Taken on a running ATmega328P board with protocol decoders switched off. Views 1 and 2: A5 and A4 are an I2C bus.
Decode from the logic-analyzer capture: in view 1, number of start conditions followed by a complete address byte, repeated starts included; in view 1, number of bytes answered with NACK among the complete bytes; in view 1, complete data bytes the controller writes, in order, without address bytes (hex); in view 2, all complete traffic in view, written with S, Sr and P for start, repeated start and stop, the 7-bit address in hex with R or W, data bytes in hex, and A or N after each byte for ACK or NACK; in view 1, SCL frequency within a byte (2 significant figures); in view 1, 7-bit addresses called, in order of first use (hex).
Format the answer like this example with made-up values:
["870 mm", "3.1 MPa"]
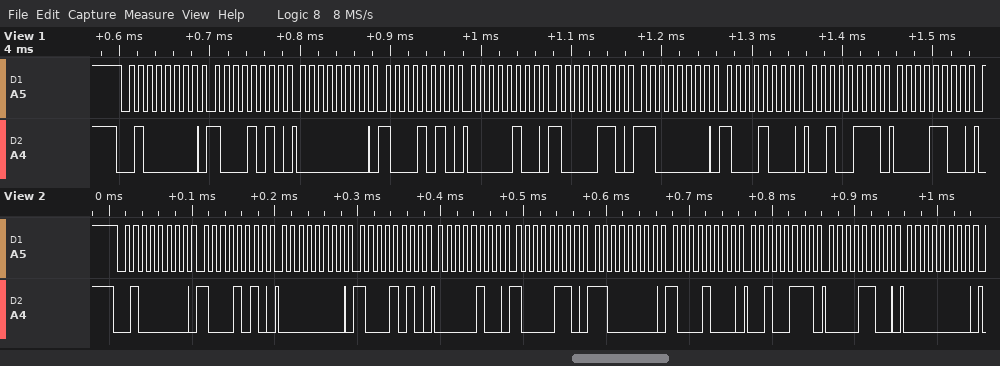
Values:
["1", "0", "8A 00 8A 04 86 C0 88 27 0C", "S 20W A 8A A 00 A 8A A 04 A 86 A C0 A 88 A 27 A 0C A 00 A", "100 kHz", "0x20"]
